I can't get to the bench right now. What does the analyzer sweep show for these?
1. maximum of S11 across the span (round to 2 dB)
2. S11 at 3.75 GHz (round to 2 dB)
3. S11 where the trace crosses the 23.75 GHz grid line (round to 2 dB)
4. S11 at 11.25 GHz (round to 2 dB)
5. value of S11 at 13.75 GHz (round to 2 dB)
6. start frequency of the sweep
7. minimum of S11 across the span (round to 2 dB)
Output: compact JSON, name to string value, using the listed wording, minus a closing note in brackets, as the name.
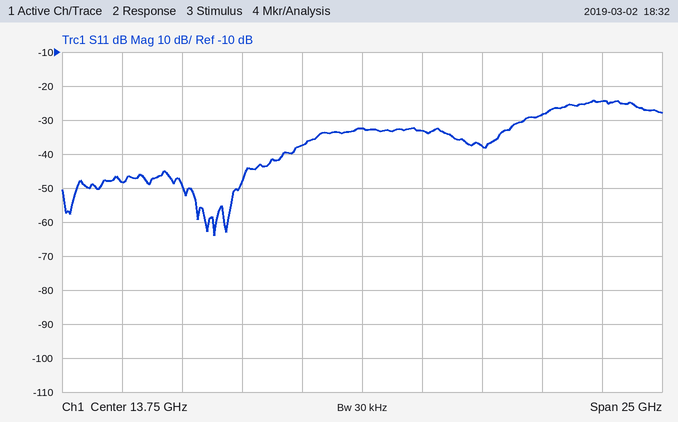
{"maximum of S11 across the span": "-24 dB", "S11 at 3.75 GHz": "-48 dB", "S11 where the trace crosses the 23.75 GHz grid line": "-24 dB", "S11 at 11.25 GHz": "-38 dB", "value of S11 at 13.75 GHz": "-32 dB", "start frequency of the sweep": "1.25 GHz", "minimum of S11 across the span": "-64 dB"}
